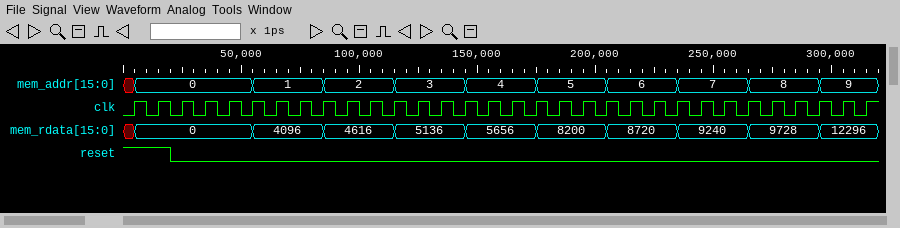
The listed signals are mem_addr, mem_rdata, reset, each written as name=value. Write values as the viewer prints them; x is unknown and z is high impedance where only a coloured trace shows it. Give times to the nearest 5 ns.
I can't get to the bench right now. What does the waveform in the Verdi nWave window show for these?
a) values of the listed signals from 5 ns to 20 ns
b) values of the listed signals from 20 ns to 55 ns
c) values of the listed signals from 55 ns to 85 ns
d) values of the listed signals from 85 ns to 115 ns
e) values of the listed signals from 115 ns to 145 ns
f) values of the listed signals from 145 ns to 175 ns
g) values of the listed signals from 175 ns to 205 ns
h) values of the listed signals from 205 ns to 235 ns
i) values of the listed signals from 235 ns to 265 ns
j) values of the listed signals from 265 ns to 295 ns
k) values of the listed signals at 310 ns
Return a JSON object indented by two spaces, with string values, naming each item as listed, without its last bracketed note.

{
  "values of the listed signals from 5 ns to 20 ns": "mem_addr=0, mem_rdata=0, reset=1",
  "values of the listed signals from 20 ns to 55 ns": "mem_addr=0, mem_rdata=0, reset=0",
  "values of the listed signals from 55 ns to 85 ns": "mem_addr=1, mem_rdata=4096, reset=0",
  "values of the listed signals from 85 ns to 115 ns": "mem_addr=2, mem_rdata=4616, reset=0",
  "values of the listed signals from 115 ns to 145 ns": "mem_addr=3, mem_rdata=5136, reset=0",
  "values of the listed signals from 145 ns to 175 ns": "mem_addr=4, mem_rdata=5656, reset=0",
  "values of the listed signals from 175 ns to 205 ns": "mem_addr=5, mem_rdata=8200, reset=0",
  "values of the listed signals from 205 ns to 235 ns": "mem_addr=6, mem_rdata=8720, reset=0",
  "values of the listed signals from 235 ns to 265 ns": "mem_addr=7, mem_rdata=9240, reset=0",
  "values of the listed signals from 265 ns to 295 ns": "mem_addr=8, mem_rdata=9728, reset=0",
  "values of the listed signals at 310 ns": "mem_addr=9, mem_rdata=12296, reset=0"
}
